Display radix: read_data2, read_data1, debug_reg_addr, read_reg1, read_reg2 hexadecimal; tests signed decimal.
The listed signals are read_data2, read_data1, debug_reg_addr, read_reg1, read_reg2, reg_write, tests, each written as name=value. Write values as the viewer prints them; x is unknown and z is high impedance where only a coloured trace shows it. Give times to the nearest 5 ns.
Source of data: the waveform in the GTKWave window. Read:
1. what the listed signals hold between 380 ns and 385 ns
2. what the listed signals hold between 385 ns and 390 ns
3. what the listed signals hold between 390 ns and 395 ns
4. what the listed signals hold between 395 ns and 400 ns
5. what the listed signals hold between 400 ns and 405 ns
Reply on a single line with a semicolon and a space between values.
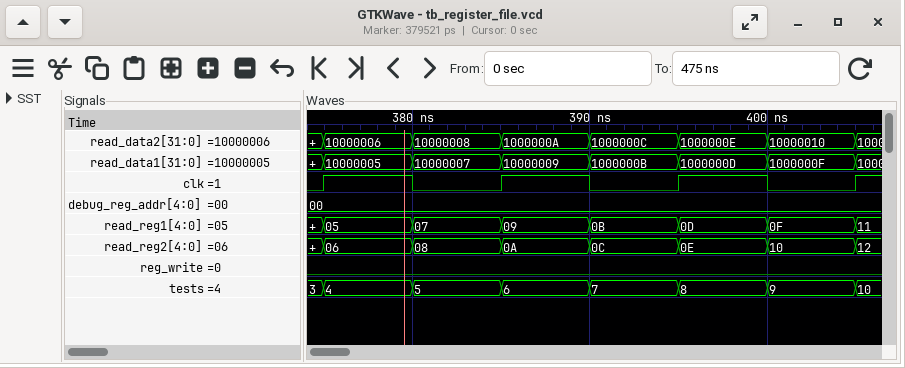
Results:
read_data2=10000008, read_data1=10000007, debug_reg_addr=00, read_reg1=07, read_reg2=08, reg_write=0, tests=5; read_data2=1000000A, read_data1=10000009, debug_reg_addr=00, read_reg1=09, read_reg2=0A, reg_write=0, tests=6; read_data2=1000000C, read_data1=1000000B, debug_reg_addr=00, read_reg1=0B, read_reg2=0C, reg_write=0, tests=7; read_data2=1000000E, read_data1=1000000D, debug_reg_addr=00, read_reg1=0D, read_reg2=0E, reg_write=0, tests=8; read_data2=10000010, read_data1=1000000F, debug_reg_addr=00, read_reg1=0F, read_reg2=10, reg_write=0, tests=9
